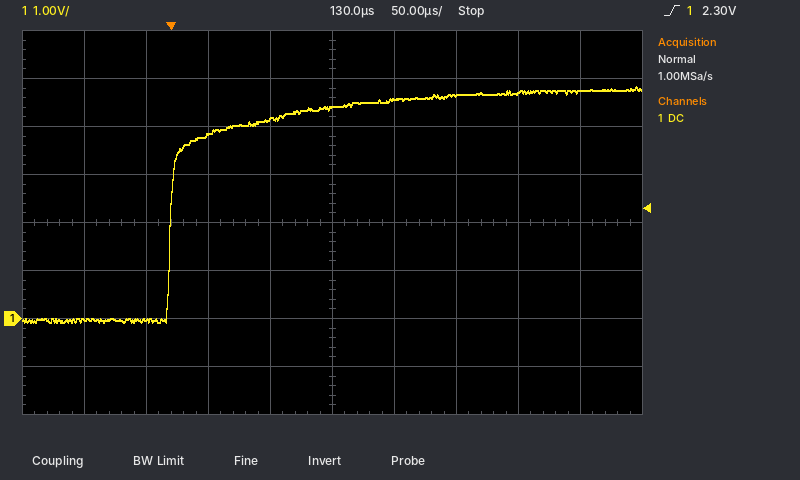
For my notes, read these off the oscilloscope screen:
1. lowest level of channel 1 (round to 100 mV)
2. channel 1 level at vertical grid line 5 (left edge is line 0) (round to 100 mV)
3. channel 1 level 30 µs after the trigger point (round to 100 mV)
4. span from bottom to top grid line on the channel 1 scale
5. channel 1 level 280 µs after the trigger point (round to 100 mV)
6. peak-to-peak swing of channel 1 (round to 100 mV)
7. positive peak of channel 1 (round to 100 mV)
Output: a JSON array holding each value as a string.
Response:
["-100 mV", "4.4 V", "3.8 V", "8 V", "4.7 V", "4.9 V", "4.8 V"]
